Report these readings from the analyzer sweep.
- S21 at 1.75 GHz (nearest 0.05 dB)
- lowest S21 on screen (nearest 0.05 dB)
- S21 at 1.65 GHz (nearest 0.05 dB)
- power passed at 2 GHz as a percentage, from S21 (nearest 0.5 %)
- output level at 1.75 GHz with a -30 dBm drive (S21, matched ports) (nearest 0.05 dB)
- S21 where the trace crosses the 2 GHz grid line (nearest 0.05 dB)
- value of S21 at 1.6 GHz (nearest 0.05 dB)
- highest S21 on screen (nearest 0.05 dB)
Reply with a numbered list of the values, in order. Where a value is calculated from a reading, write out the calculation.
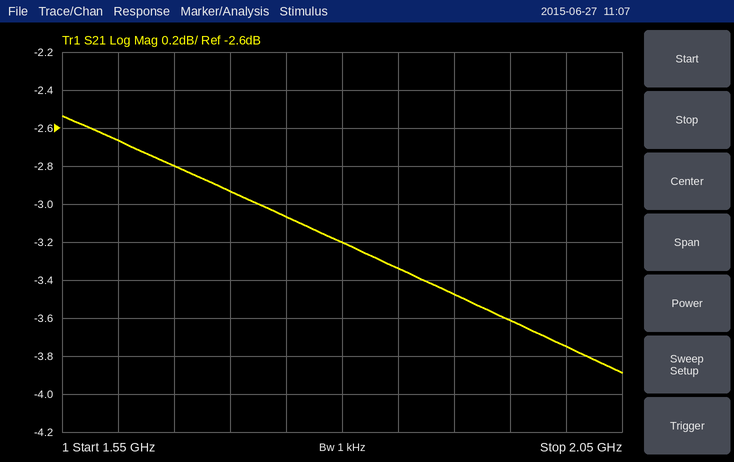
1. -3.05 dB
2. -3.90 dB
3. -2.80 dB
4. 10^(-3.75/10) ≈ 42.2 %, so 42.0 % to the nearest 0.5 %
5. -30 dBm + (-3.05 dB) = -33.05 dBm
6. -3.75 dB
7. -2.65 dB
8. -2.55 dB
